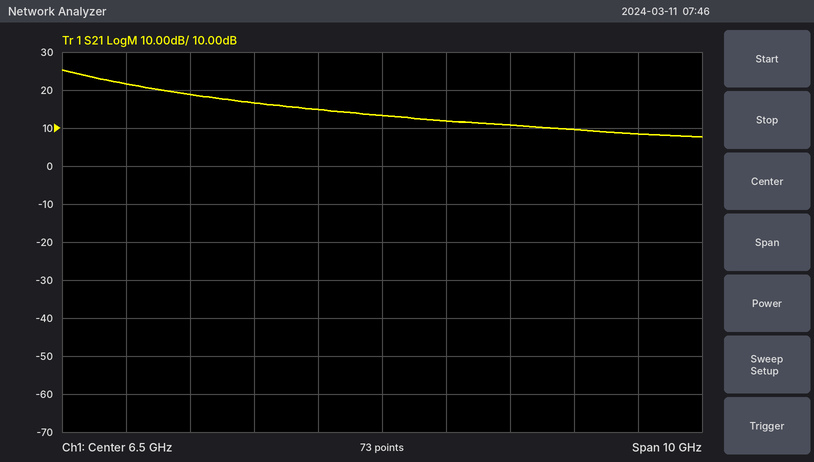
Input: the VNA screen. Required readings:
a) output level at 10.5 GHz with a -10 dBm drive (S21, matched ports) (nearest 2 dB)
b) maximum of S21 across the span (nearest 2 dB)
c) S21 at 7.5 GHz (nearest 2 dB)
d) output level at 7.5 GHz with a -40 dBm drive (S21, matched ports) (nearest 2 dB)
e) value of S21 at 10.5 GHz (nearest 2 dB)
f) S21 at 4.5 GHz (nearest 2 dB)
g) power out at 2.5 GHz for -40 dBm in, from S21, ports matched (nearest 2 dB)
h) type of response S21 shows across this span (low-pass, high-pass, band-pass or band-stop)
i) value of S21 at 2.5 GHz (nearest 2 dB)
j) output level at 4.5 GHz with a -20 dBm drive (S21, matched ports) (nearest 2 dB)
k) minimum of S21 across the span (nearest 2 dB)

-2 dBm
26 dB
12 dB
-28 dBm
8 dB
16 dB
-18 dBm
low-pass
22 dB
-4 dBm
8 dB
